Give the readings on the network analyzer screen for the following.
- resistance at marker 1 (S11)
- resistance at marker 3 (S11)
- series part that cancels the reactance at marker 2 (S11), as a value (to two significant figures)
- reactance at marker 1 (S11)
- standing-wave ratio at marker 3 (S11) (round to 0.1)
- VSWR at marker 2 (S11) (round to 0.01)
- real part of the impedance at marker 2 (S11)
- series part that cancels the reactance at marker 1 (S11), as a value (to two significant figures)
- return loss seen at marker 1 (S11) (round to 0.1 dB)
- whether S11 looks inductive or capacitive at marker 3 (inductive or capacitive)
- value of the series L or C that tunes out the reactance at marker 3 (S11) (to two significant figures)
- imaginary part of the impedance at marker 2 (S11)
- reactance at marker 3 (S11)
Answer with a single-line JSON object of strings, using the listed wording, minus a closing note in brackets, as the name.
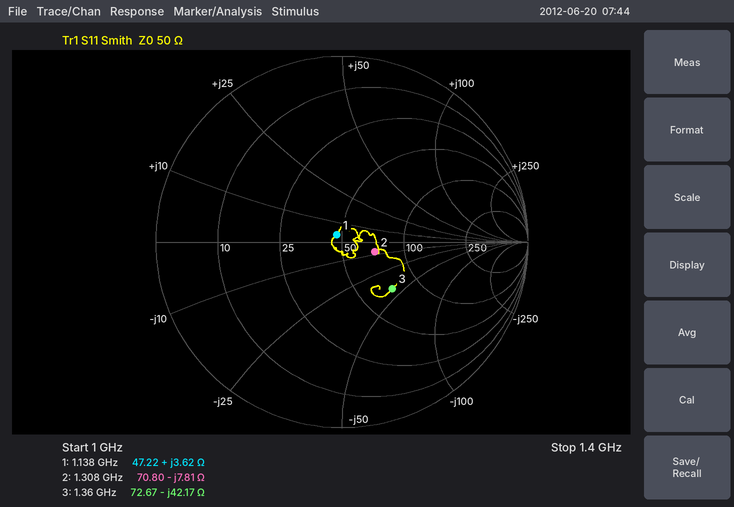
{"resistance at marker 1": "47.22 Ω", "resistance at marker 3": "72.67 Ω", "series part that cancels the reactance at marker 2 (S11), as a value": "950 pH", "reactance at marker 1": "+3.62 Ω", "standing-wave ratio at marker 3 (S11)": "2.2", "VSWR at marker 2 (S11)": "1.45", "real part of the impedance at marker 2": "70.80 Ω", "series part that cancels the reactance at marker 1 (S11), as a value": "39 pF", "return loss seen at marker 1 (S11)": "26.6 dB", "whether S11 looks inductive or capacitive at marker 3": "capacitive", "value of the series L or C that tunes out the reactance at marker 3 (S11)": "4.9 nH", "imaginary part of the impedance at marker 2": "-7.81 Ω", "reactance at marker 3": "-42.17 Ω"}
